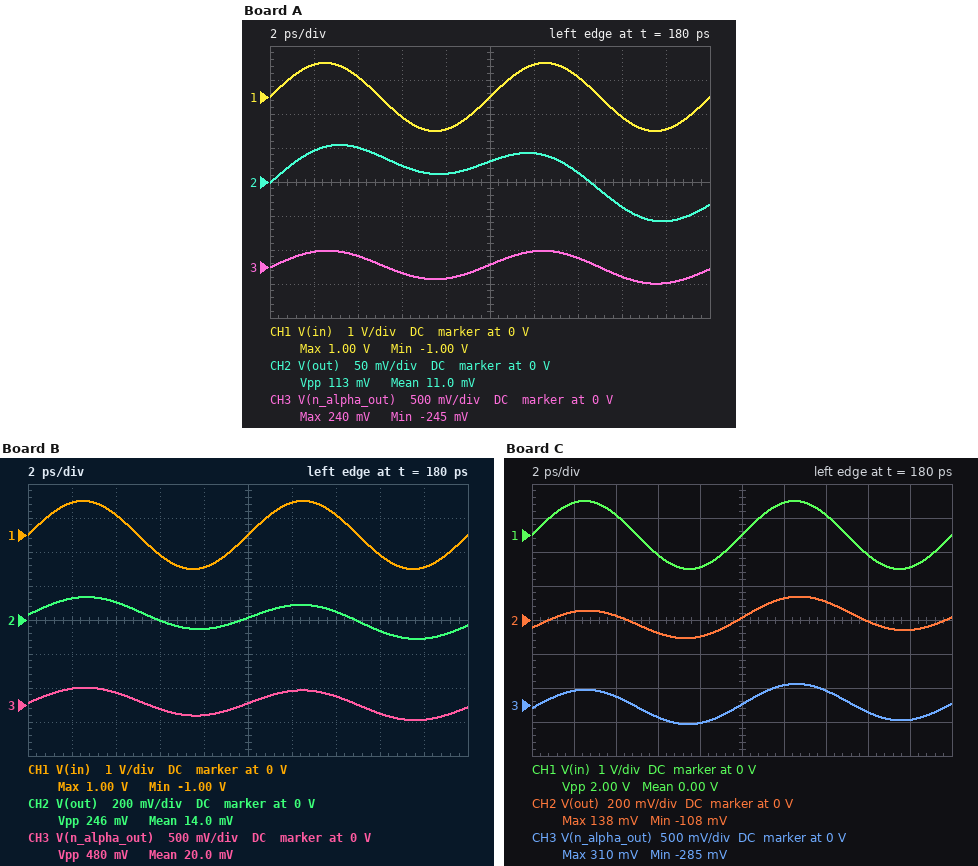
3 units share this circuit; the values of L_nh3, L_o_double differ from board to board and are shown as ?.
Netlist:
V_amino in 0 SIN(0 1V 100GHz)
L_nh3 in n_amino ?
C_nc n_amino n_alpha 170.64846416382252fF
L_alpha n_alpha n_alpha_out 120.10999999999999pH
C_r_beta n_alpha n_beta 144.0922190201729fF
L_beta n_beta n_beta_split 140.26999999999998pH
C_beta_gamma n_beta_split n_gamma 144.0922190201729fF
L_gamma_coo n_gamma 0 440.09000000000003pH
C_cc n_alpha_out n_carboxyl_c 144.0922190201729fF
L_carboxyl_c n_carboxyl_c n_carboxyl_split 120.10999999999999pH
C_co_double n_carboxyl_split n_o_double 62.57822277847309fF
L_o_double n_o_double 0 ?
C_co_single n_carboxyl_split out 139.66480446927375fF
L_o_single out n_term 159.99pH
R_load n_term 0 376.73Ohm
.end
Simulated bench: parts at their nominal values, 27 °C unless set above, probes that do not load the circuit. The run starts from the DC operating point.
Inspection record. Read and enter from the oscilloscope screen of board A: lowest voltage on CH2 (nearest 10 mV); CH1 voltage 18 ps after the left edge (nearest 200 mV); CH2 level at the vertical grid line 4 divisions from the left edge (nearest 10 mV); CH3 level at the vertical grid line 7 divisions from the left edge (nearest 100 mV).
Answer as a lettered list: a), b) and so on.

a) -60 mV
b) -1.0 V
c) 10 mV
d) 100 mV
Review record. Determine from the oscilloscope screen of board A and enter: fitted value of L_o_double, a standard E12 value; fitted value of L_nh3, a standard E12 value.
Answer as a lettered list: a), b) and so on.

a) 56 pH
b) 220 pH
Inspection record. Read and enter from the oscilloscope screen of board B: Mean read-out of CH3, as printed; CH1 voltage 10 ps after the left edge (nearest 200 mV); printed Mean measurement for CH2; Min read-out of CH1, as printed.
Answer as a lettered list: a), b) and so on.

a) 20.0 mV
b) 0 V
c) 14.0 mV
d) -1.00 V
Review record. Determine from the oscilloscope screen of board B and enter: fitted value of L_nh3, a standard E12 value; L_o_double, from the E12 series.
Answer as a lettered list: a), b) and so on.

a) 390 pH
b) 120 pH
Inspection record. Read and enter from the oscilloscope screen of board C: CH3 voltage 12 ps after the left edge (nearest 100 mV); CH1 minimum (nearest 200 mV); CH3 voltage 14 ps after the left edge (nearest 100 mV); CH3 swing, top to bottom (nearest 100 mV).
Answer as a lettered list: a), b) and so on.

a) 300 mV
b) -1.0 V
c) 200 mV
d) 600 mV
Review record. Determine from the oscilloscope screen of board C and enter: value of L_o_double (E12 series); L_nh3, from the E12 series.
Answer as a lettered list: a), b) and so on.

a) 100 pH
b) 220 pH
